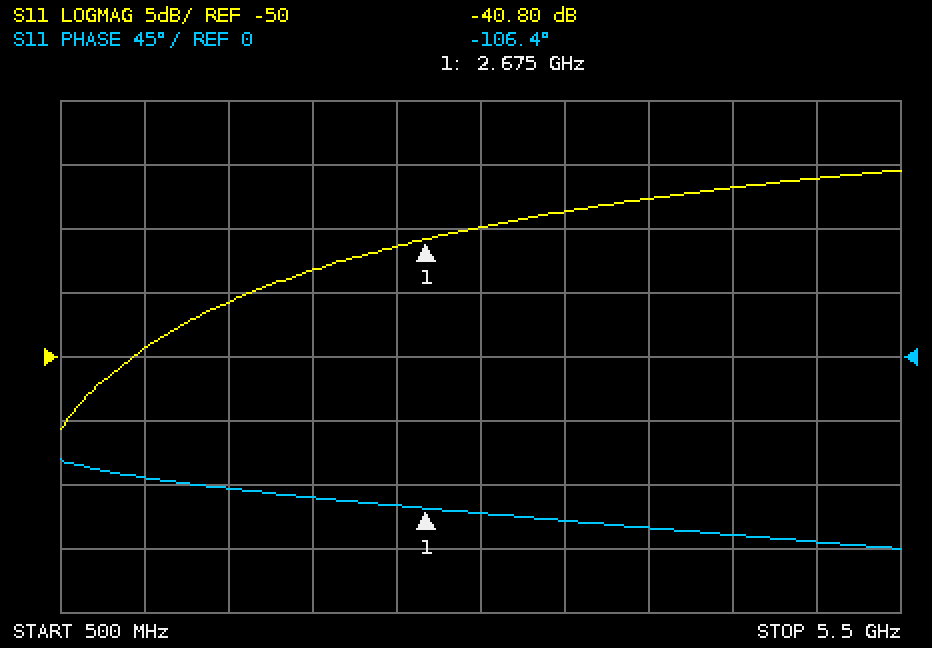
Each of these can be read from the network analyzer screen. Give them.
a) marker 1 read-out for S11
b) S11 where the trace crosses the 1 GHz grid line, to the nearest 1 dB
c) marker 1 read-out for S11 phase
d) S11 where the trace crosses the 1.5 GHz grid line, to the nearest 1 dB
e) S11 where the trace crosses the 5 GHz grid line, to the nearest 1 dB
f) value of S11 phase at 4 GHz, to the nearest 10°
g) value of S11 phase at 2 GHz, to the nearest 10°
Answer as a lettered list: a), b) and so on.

a) -40.80 dB
b) -49 dB
c) -106.4°
d) -46 dB
e) -36 dB
f) -120°
g) -100°
